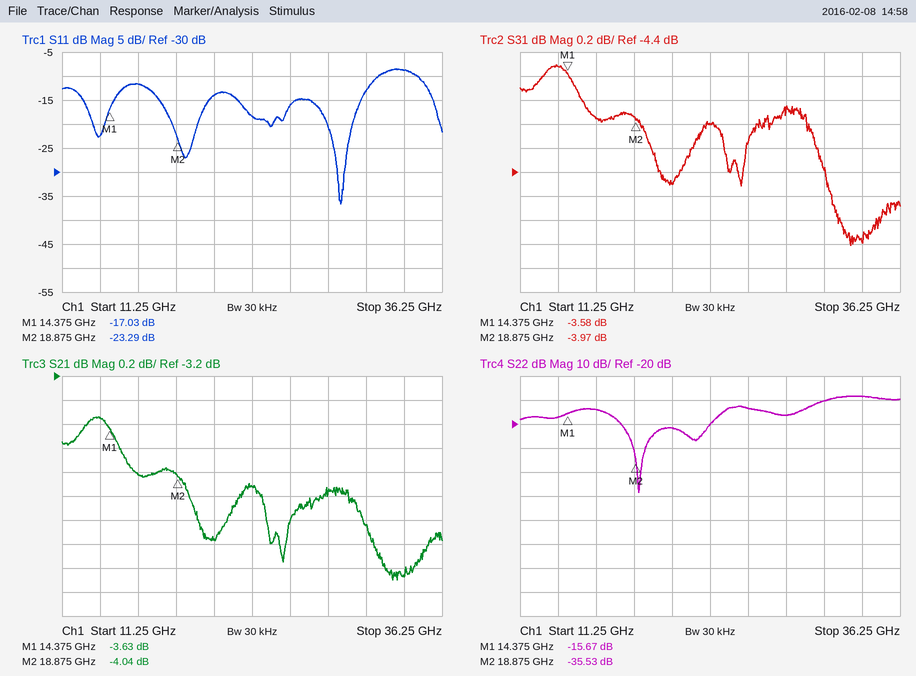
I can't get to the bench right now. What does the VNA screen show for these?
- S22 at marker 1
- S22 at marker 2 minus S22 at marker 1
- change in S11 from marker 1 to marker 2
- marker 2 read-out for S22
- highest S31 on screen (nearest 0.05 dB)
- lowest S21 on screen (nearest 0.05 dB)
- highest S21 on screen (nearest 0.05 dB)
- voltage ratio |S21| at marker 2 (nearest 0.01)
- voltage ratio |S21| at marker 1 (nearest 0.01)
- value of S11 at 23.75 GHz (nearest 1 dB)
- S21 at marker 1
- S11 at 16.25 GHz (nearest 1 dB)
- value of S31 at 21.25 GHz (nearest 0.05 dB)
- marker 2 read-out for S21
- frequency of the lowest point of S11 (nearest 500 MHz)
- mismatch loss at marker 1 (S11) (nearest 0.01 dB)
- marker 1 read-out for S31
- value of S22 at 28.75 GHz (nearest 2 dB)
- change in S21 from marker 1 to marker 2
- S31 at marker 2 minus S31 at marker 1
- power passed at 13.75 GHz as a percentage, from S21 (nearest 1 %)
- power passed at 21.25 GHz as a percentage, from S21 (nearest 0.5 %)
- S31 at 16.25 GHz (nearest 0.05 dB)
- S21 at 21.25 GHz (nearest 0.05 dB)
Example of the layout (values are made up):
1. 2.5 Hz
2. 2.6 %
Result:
1. -15.67 dB
2. -19.86 dB
3. -6.26 dB
4. -35.53 dB
5. -3.50 dB
6. -4.90 dB
7. -3.55 dB
8. 0.63
9. 0.66
10. -18 dB
11. -3.63 dB
12. -12 dB
13. -4.50 dB
14. -4.04 dB
15. 29.5 GHz
16. 0.09 dB
17. -3.58 dB
18. -16 dB
19. -0.41 dB
20. -0.39 dB
21. 44 %
22. 35.0 %
23. -3.95 dB
24. -4.55 dB
